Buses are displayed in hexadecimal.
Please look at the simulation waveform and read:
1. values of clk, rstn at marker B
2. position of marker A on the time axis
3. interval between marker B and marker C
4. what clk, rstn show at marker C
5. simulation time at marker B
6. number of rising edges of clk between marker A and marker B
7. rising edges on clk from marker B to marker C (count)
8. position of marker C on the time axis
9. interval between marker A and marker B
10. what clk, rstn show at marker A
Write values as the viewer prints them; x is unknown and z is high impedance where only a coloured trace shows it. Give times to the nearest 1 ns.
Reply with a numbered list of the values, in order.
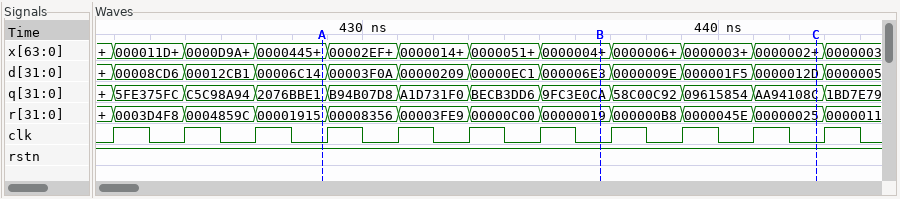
1. clk=0, rstn=1
2. 429 ns
3. 6 ns
4. clk=0, rstn=1
5. 437 ns
6. 4
7. 3
8. 443 ns
9. 8 ns
10. clk=0, rstn=1
